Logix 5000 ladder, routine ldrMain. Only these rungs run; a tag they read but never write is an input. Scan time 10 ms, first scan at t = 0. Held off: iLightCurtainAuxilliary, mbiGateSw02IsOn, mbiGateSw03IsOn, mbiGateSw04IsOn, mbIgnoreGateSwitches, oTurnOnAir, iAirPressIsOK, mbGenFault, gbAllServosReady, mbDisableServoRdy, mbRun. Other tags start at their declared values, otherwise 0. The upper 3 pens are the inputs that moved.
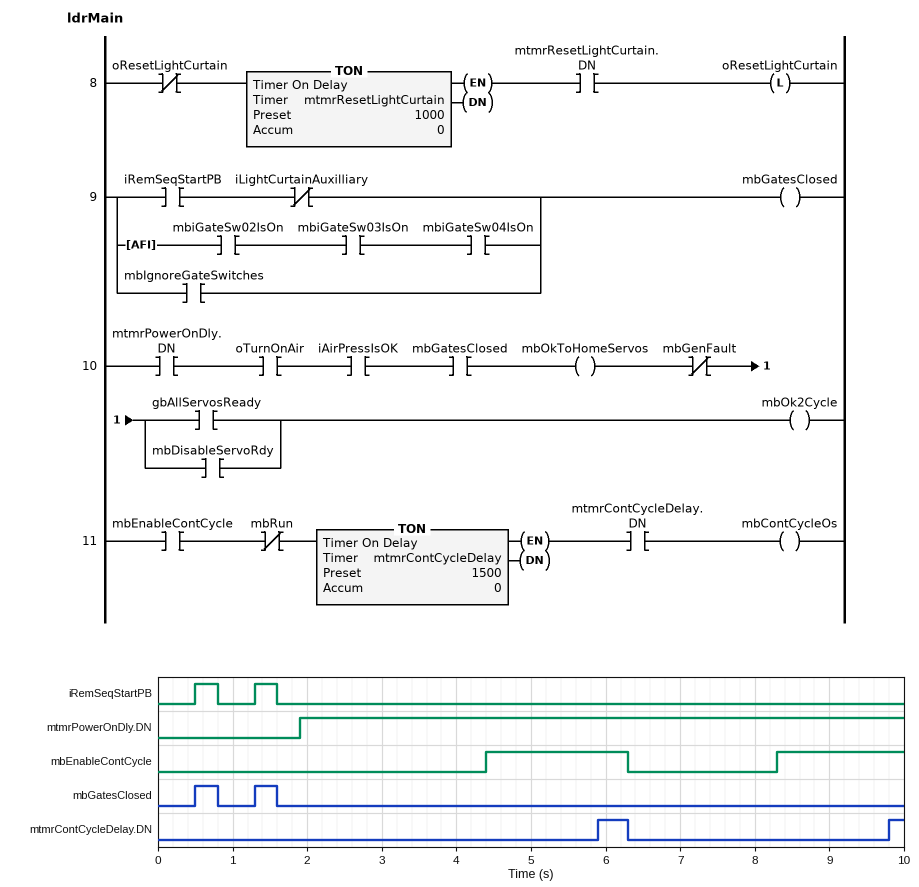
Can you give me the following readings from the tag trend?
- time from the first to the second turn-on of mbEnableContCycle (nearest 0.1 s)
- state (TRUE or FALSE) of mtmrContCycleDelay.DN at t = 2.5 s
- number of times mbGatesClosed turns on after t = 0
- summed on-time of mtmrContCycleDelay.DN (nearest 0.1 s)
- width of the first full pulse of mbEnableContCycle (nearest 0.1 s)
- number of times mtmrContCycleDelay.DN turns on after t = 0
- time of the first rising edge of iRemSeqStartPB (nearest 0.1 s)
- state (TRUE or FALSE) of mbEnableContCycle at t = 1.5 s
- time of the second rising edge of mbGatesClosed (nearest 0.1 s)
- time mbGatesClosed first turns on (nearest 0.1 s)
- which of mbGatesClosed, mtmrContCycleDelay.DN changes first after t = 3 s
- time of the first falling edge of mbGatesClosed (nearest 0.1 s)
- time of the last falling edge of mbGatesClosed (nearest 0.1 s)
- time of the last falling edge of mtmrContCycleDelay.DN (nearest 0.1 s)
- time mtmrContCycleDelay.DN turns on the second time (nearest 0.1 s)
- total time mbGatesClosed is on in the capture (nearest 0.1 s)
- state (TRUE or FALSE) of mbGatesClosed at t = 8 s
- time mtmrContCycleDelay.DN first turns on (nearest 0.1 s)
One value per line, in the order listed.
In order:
3.9 s
FALSE
2
0.6 s
1.9 s
2
0.5 s
FALSE
1.3 s
0.5 s
mtmrContCycleDelay.DN
0.8 s
1.6 s
6.3 s
9.8 s
0.6 s
FALSE
5.9 s
